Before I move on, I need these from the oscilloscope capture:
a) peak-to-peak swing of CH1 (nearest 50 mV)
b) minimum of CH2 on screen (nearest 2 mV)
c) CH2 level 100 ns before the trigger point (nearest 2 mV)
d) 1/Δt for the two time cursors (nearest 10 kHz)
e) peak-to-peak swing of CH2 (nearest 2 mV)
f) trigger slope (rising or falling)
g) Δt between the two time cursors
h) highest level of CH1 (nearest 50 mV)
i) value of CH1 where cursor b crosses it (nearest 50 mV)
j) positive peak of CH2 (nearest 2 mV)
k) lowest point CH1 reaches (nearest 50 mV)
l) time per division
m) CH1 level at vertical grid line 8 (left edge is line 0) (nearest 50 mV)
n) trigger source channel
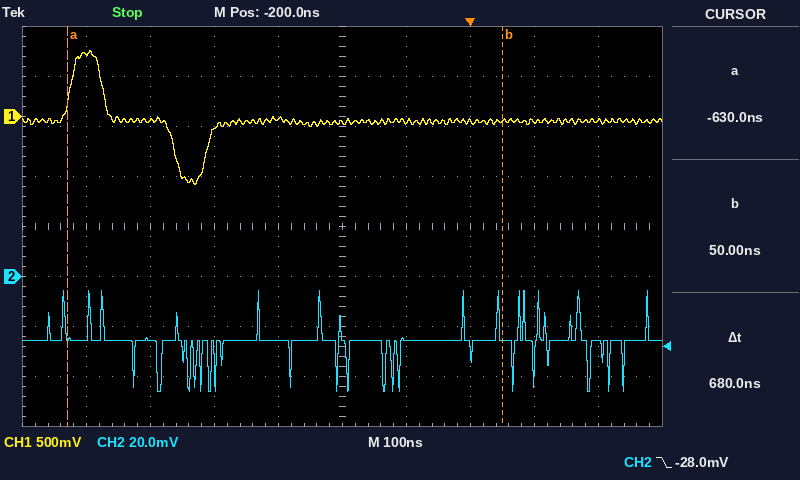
1.35 V
-46 mV
-26 mV
1.47 MHz
40 mV
falling
680 ns
650 mV
-50 mV
-6 mV
-700 mV
100 ns
-50 mV
CH2
